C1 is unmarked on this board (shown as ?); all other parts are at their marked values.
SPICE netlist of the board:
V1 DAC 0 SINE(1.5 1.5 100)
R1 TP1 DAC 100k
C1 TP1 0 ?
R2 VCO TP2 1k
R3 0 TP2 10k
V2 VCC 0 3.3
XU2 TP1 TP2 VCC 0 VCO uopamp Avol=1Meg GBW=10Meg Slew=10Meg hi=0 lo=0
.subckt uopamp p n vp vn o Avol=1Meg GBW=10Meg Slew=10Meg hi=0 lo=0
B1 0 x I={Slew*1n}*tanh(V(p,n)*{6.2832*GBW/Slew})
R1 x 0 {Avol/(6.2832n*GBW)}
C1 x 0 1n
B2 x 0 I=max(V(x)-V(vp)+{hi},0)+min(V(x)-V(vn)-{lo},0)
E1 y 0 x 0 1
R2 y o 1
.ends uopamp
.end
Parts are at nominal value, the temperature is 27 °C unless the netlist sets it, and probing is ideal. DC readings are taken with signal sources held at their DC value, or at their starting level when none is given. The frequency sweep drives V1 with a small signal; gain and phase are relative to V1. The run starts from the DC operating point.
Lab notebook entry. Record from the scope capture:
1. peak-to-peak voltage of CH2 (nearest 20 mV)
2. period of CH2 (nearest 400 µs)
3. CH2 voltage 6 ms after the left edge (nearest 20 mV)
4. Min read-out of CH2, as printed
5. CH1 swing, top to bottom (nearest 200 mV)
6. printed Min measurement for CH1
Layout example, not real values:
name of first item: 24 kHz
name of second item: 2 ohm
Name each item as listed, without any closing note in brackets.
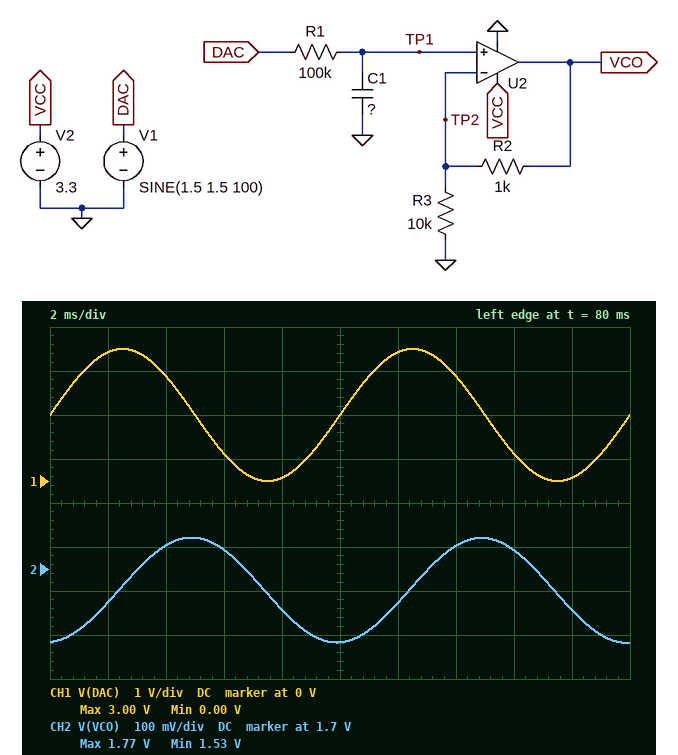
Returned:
peak-to-peak voltage of CH2: 240 mV
period of CH2: 10.0 ms
CH2 voltage 6 ms after the left edge: 1.74 V
Min read-out of CH2, as printed: 1.53 V
CH1 swing, top to bottom: 3.0 V
printed Min measurement for CH1: 0.00 V
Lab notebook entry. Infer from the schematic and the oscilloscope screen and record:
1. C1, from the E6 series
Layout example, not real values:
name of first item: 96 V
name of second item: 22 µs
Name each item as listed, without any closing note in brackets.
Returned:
C1, from the E6 series: 220 nF
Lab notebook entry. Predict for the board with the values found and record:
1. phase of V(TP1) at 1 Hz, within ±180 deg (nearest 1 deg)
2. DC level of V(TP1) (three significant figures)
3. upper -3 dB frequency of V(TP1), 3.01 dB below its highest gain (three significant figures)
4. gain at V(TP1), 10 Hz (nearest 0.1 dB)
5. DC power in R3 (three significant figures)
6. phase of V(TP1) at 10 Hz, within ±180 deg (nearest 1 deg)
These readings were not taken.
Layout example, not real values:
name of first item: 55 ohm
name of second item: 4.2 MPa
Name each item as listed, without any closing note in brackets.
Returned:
phase of V(TP1) at 1 Hz, within ±180 deg: -8 deg
DC level of V(TP1): 1.50 V
upper -3 dB frequency of V(TP1), 3.01 dB below its highest gain: 7.23 Hz
gain at V(TP1), 10 Hz: -4.6 dB
DC power in R3: 225 µW
phase of V(TP1) at 10 Hz, within ±180 deg: -54 deg
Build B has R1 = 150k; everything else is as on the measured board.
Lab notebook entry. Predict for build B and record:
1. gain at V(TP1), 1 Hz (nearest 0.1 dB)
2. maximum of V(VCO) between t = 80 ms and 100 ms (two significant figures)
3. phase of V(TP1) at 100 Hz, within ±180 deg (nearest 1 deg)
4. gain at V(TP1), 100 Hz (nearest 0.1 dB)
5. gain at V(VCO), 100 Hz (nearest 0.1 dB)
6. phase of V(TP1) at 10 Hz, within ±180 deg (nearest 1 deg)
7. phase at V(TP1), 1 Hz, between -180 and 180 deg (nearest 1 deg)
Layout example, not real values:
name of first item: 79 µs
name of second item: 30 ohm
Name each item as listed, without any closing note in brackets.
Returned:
gain at V(TP1), 1 Hz: -0.2 dB
maximum of V(VCO) between t = 80 ms and 100 ms: 1.7 V
phase of V(TP1) at 100 Hz, within ±180 deg: -87 deg
gain at V(TP1), 100 Hz: -26.3 dB
gain at V(VCO), 100 Hz: -25.5 dB
phase of V(TP1) at 10 Hz, within ±180 deg: -64 deg
phase at V(TP1), 1 Hz, between -180 and 180 deg: -12 deg
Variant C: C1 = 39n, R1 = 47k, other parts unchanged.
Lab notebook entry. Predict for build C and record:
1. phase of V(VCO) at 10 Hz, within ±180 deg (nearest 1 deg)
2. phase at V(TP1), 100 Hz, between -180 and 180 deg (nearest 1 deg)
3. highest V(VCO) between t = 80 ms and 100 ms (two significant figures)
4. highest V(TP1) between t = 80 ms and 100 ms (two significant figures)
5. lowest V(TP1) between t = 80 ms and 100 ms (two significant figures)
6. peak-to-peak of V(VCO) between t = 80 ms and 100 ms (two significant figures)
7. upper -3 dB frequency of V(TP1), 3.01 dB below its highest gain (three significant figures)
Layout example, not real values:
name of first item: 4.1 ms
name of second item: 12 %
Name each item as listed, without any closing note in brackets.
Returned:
phase of V(VCO) at 10 Hz, within ±180 deg: -7 deg
phase at V(TP1), 100 Hz, between -180 and 180 deg: -49 deg
highest V(VCO) between t = 80 ms and 100 ms: 2.7 V
highest V(TP1) between t = 80 ms and 100 ms: 2.5 V
lowest V(TP1) between t = 80 ms and 100 ms: 520 mV
peak-to-peak of V(VCO) between t = 80 ms and 100 ms: 2.2 V
upper -3 dB frequency of V(TP1), 3.01 dB below its highest gain: 86.8 Hz
